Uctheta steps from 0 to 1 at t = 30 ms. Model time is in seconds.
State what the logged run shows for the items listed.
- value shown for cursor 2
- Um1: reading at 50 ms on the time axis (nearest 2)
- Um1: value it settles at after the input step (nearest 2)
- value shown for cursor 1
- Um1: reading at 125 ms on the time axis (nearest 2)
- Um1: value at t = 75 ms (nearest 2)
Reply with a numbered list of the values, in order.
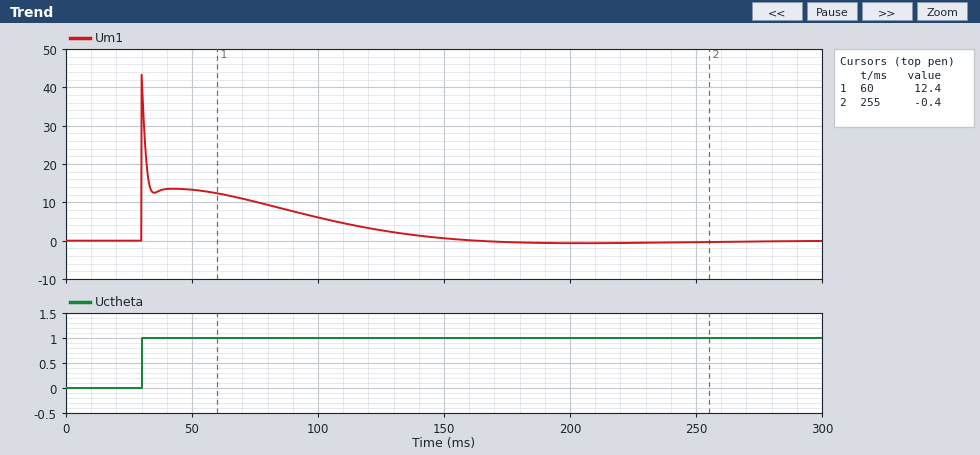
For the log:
1. -0.4
2. 14
3. 0
4. 12.4
5. 2
6. 10
